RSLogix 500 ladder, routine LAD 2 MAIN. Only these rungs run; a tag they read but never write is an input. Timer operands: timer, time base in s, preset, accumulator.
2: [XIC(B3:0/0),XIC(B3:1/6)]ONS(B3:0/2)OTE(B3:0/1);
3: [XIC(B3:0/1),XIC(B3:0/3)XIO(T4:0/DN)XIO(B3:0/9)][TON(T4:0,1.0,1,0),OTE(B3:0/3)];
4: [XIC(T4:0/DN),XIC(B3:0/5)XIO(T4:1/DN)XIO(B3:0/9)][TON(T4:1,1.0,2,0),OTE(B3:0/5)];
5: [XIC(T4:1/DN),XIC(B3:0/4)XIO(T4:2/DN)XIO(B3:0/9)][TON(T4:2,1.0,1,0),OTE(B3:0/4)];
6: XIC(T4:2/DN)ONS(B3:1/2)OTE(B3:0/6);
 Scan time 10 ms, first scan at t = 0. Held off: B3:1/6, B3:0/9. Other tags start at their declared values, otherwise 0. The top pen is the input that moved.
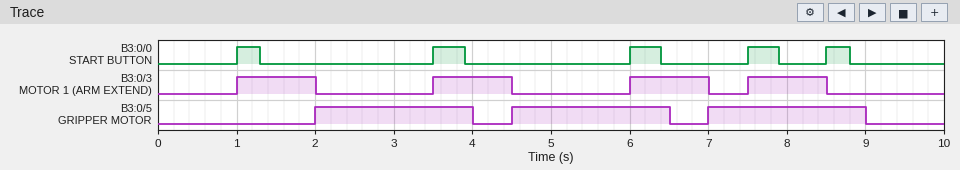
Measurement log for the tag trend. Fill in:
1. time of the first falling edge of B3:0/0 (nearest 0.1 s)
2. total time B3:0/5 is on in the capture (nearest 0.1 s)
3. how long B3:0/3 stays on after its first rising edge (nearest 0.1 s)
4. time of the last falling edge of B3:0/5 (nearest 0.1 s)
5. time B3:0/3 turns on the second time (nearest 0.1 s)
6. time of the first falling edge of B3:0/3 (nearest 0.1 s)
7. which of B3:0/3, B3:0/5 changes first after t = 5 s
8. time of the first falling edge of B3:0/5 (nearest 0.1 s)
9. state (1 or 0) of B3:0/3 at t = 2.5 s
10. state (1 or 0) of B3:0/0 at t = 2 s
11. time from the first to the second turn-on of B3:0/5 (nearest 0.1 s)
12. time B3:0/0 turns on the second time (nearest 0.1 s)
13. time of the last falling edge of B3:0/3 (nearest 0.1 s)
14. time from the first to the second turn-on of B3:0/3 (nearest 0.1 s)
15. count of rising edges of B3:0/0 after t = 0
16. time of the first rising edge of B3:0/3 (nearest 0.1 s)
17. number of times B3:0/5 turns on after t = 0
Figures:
1.3 s
6.0 s
1.0 s
9.0 s
3.5 s
2.0 s
B3:0/3
4.0 s
0
0
2.5 s
3.5 s
8.5 s
2.5 s
5
1.0 s
3
